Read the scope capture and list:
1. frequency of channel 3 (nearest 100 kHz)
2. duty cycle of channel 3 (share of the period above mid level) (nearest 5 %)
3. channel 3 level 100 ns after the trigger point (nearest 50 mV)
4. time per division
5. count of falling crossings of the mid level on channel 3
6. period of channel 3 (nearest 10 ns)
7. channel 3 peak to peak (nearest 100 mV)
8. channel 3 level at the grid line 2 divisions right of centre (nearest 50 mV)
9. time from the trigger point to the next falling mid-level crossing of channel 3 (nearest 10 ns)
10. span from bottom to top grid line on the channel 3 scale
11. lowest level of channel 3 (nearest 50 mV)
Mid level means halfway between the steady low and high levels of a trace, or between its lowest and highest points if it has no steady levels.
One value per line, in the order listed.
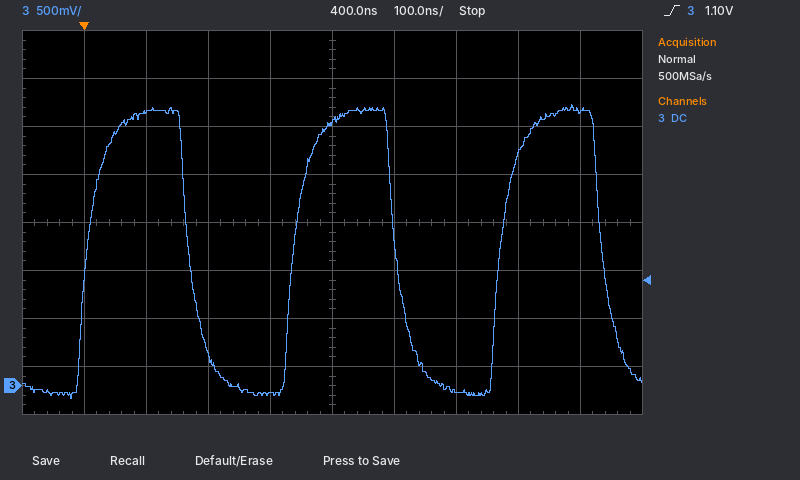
3.0 MHz
50 %
2.85 V
100 ns
3
330 ns
3.10 V
-50 mV
170 ns
4 V
-150 mV
